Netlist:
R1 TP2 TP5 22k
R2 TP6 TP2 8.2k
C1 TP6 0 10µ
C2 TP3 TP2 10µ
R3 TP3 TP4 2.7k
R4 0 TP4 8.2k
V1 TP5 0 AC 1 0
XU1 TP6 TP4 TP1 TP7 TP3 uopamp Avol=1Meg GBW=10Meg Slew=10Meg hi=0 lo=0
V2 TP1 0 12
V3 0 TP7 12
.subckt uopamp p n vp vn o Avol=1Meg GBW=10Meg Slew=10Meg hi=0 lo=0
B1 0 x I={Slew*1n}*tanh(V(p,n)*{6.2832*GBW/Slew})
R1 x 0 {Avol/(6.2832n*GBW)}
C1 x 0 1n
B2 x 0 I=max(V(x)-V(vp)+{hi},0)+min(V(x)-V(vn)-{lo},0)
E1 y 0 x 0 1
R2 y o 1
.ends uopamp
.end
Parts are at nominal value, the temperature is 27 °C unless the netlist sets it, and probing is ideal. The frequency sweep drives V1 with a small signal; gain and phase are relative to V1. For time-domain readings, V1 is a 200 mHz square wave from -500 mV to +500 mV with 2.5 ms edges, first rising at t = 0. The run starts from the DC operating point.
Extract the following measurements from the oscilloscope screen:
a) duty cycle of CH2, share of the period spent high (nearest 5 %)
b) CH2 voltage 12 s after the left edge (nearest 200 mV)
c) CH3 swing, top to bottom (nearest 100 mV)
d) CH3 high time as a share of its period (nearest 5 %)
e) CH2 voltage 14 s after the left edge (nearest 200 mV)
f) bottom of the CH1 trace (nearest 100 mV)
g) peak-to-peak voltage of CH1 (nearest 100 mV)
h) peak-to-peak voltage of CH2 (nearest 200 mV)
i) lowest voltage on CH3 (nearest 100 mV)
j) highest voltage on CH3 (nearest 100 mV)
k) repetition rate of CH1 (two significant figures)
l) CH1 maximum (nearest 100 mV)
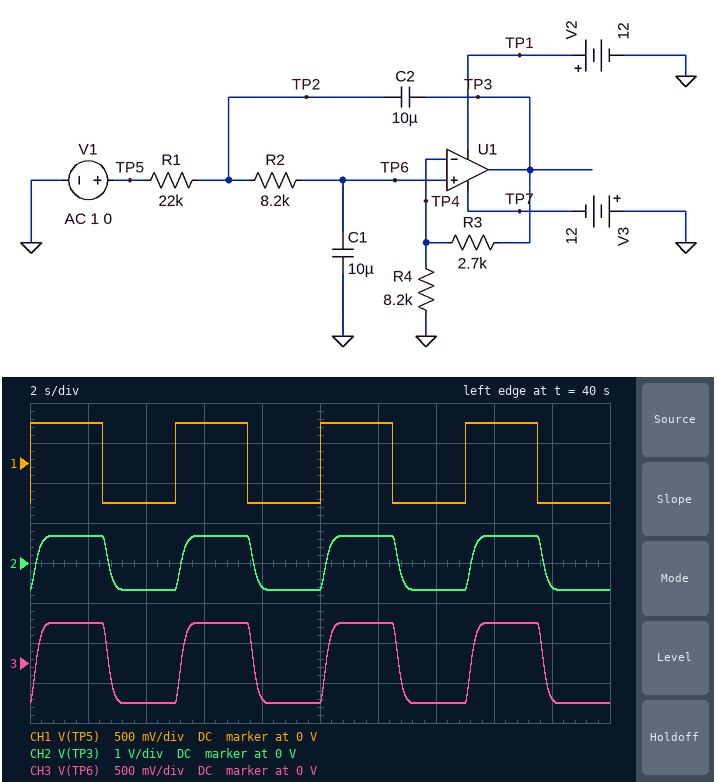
50 %
600 mV
1.0 V
50 %
-600 mV
-500 mV
1.0 V
1.4 V
-500 mV
500 mV
200 mHz
500 mV
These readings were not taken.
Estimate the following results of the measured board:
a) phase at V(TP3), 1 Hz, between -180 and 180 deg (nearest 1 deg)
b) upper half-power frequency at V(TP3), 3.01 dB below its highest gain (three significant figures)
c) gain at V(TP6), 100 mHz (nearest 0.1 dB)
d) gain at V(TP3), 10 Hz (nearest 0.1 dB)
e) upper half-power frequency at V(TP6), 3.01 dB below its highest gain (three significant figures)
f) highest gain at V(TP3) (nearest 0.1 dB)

-79 deg
948 mHz
0 dB
-34.6 dB
948 mHz
2.5 dB
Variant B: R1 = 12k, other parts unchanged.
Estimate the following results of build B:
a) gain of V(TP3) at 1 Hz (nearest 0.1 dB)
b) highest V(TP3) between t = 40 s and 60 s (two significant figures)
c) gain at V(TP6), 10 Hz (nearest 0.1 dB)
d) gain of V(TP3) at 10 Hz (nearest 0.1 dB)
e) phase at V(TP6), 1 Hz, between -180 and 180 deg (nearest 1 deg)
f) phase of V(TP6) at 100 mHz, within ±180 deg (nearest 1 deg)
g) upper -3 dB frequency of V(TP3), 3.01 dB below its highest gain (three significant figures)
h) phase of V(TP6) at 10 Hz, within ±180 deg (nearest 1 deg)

1.0 dB
680 mV
-31.9 dB
-29.4 dB
-59 deg
-6 deg
1.36 Hz
-165 deg
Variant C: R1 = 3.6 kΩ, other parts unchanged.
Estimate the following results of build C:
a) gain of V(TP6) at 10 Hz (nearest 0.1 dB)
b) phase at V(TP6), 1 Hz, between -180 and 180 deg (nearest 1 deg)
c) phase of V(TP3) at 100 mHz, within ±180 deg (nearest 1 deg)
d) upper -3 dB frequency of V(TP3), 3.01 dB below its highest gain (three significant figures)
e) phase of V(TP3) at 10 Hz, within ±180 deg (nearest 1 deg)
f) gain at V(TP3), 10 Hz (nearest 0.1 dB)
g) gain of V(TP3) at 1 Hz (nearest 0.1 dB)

-22.0 dB
-37 deg
-4 deg
1.95 Hz
-148 deg
-19.5 dB
1.6 dB
